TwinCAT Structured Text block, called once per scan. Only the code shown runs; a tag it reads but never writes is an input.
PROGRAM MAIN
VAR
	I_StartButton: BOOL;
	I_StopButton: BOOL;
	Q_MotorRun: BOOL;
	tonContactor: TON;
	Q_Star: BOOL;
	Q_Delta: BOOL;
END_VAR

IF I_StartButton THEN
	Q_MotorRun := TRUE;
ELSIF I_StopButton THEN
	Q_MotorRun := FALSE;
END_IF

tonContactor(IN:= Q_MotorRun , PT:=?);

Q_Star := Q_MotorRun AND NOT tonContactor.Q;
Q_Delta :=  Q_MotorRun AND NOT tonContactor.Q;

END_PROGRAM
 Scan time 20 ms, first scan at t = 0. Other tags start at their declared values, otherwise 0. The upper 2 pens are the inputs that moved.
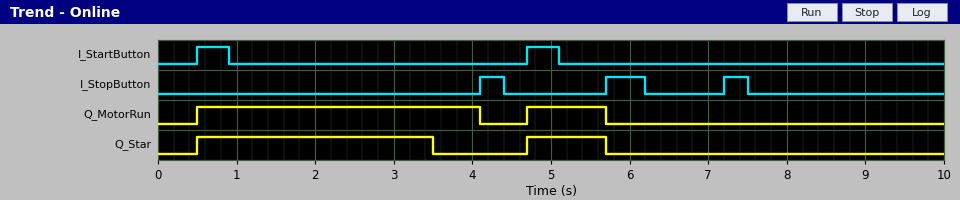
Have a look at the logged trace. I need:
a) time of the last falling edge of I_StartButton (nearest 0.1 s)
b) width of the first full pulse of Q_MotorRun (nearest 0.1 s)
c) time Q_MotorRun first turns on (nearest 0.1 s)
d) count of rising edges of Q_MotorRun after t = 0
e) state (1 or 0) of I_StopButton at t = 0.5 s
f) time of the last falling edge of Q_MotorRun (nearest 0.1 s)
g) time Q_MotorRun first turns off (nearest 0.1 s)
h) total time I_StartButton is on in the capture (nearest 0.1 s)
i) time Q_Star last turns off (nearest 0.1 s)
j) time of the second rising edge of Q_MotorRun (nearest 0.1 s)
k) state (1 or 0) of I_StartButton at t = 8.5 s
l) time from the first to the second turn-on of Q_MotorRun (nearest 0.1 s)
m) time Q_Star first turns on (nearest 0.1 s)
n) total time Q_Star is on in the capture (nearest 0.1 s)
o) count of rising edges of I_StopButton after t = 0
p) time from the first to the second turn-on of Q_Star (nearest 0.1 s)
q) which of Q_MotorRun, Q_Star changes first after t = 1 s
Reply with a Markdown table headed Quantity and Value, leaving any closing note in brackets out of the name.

| Quantity | Value |
|---|---|
| time of the last falling edge of I_StartButton | 5.1 s |
| width of the first full pulse of Q_MotorRun | 3.6 s |
| time Q_MotorRun first turns on | 0.5 s |
| count of rising edges of Q_MotorRun after t = 0 | 2 |
| state (1 or 0) of I_StopButton at t = 0.5 s | 0 |
| time of the last falling edge of Q_MotorRun | 5.7 s |
| time Q_MotorRun first turns off | 4.1 s |
| total time I_StartButton is on in the capture | 0.8 s |
| time Q_Star last turns off | 5.7 s |
| time of the second rising edge of Q_MotorRun | 4.7 s |
| state (1 or 0) of I_StartButton at t = 8.5 s | 0 |
| time from the first to the second turn-on of Q_MotorRun | 4.2 s |
| time Q_Star first turns on | 0.5 s |
| total time Q_Star is on in the capture | 4.0 s |
| count of rising edges of I_StopButton after t = 0 | 3 |
| time from the first to the second turn-on of Q_Star | 4.2 s |
| which of Q_MotorRun, Q_Star changes first after t = 1 s | Q_Star |
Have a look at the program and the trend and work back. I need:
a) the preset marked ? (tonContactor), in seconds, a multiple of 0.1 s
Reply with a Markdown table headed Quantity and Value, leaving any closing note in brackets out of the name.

| Quantity | Value |
|---|---|
| the preset marked ? (tonContactor), in seconds, a multiple of 0.1 s | 3.0 s |
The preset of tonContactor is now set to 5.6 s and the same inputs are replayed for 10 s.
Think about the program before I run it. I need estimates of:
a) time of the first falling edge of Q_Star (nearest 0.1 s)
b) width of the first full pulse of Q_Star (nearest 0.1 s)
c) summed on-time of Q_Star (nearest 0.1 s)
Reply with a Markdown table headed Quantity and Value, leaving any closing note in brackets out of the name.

| Quantity | Value |
|---|---|
| time of the first falling edge of Q_Star | 4.1 s |
| width of the first full pulse of Q_Star | 3.6 s |
| summed on-time of Q_Star | 4.6 s |
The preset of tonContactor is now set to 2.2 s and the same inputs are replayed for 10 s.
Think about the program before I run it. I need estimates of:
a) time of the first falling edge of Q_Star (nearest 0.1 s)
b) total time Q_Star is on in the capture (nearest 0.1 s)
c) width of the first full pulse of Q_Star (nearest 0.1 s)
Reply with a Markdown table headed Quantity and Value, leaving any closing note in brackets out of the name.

| Quantity | Value |
|---|---|
| time of the first falling edge of Q_Star | 2.7 s |
| total time Q_Star is on in the capture | 3.2 s |
| width of the first full pulse of Q_Star | 2.2 s |
